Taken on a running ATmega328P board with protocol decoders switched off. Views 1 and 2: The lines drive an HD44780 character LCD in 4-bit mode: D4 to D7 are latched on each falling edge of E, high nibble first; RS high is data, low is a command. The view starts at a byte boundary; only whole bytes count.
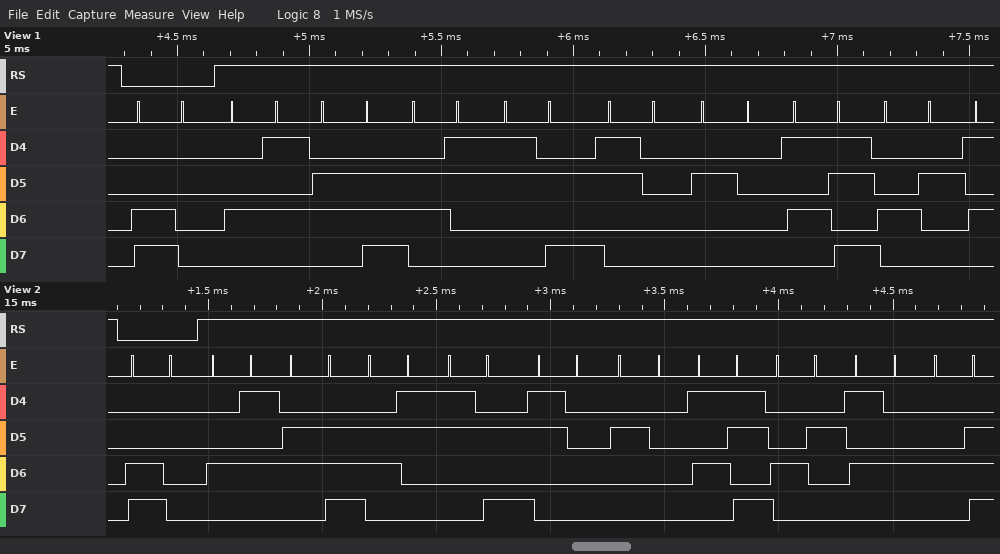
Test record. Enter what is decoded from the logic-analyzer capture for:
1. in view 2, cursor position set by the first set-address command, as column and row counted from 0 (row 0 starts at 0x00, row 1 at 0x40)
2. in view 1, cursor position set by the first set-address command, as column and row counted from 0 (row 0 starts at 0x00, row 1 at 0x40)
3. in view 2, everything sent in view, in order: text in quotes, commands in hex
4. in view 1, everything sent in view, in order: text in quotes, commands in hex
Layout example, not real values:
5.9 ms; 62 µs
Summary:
column 0, row 1; column 0, row 1; 0xC0 "Enc:0 [BTN"; 0xC0 "Enc:0 [B"
